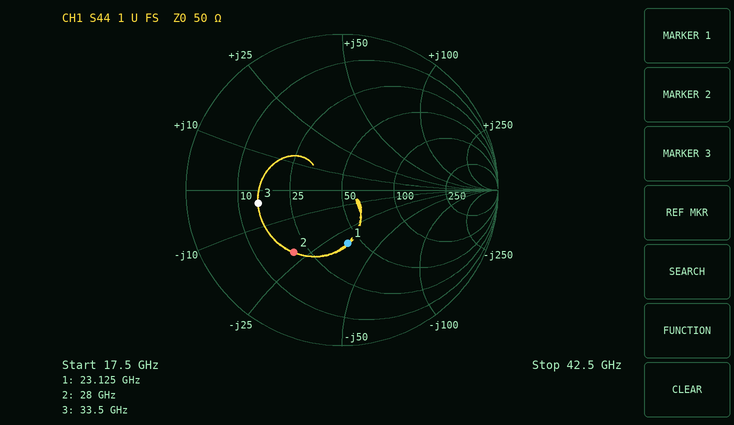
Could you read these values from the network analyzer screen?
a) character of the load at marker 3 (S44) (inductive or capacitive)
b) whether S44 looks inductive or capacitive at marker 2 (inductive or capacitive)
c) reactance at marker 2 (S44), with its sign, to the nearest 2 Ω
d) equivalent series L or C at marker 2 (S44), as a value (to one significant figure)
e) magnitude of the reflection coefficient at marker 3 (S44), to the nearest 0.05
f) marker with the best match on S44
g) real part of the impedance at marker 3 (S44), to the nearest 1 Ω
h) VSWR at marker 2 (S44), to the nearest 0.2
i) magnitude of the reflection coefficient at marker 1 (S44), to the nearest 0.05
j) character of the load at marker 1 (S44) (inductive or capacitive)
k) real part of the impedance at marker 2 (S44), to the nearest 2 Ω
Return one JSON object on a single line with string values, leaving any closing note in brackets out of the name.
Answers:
{"character of the load at marker 3 (S44)": "capacitive", "whether S44 looks inductive or capacitive at marker 2": "capacitive", "reactance at marker 2 (S44), with its sign, to the nearest 2 Ω": "-22 Ω", "equivalent series L or C at marker 2 (S44), as a value": "300 fF", "magnitude of the reflection coefficient at marker 3 (S44), to the nearest 0.05": "0.55", "marker with the best match on S44": "marker 1", "real part of the impedance at marker 3 (S44), to the nearest 1 Ω": "15 Ω", "VSWR at marker 2 (S44), to the nearest 0.2": "3.0", "magnitude of the reflection coefficient at marker 1 (S44), to the nearest 0.05": "0.35", "character of the load at marker 1 (S44)": "capacitive", "real part of the impedance at marker 2 (S44), to the nearest 2 Ω": "20 Ω"}
